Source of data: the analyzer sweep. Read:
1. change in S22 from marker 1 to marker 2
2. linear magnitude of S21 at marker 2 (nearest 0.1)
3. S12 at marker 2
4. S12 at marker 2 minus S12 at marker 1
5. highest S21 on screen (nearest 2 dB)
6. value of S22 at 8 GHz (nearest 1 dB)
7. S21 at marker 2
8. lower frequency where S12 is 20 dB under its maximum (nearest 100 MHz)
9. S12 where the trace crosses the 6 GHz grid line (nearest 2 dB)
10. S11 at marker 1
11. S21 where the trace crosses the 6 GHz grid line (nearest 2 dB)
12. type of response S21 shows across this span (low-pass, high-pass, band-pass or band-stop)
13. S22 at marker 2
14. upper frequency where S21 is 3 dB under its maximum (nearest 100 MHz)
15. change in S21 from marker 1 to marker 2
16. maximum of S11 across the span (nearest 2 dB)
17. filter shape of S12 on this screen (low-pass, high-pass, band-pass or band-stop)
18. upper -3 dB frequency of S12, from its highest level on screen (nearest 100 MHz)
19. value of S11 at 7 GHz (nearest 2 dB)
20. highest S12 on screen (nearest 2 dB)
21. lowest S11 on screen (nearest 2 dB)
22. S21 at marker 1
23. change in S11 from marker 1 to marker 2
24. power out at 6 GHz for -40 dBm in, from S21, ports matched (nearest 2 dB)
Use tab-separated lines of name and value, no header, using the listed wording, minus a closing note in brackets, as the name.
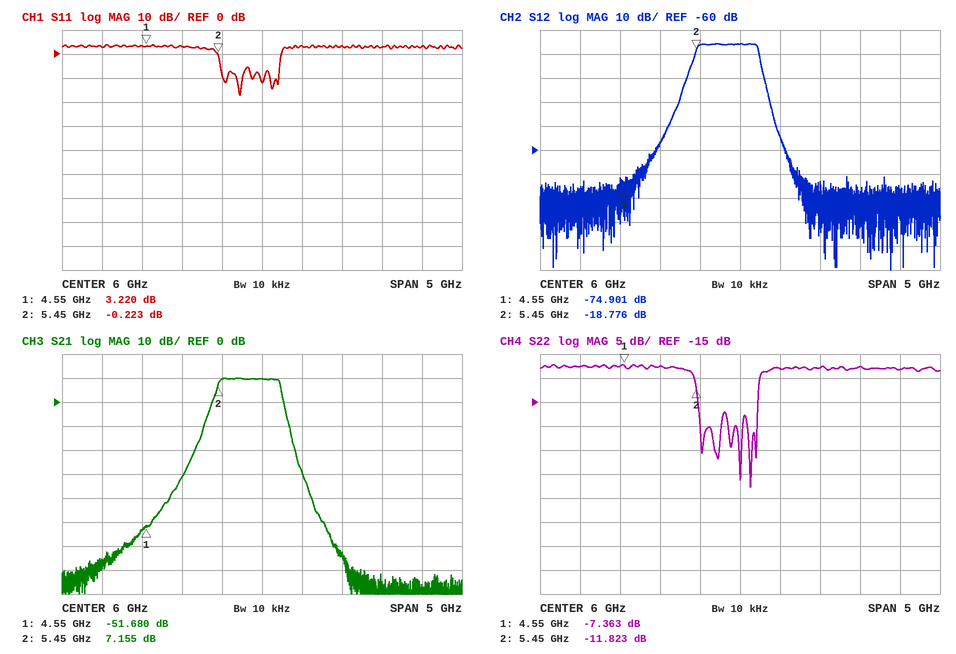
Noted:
change in S22 from marker 1 to marker 2	-4.460 dB
linear magnitude of S21 at marker 2	2.3
S12 at marker 2	-18.776 dB
S12 at marker 2 minus S12 at marker 1	56.125 dB
highest S21 on screen	10 dB
value of S22 at 8 GHz	-8 dB
S21 at marker 2	7.155 dB
lower frequency where S12 is 20 dB under its maximum	5.3 GHz
S12 where the trace crosses the 6 GHz grid line	-16 dB
S11 at marker 1	3.220 dB
S21 where the trace crosses the 6 GHz grid line	10 dB
type of response S21 shows across this span	band-pass
S22 at marker 2	-11.823 dB
upper frequency where S21 is 3 dB under its maximum	6.2 GHz
change in S21 from marker 1 to marker 2	58.835 dB
maximum of S11 across the span	4 dB
filter shape of S12 on this screen	band-pass
upper -3 dB frequency of S12, from its highest level on screen	6.2 GHz
value of S11 at 7 GHz	4 dB
highest S12 on screen	-16 dB
lowest S11 on screen	-18 dB
S21 at marker 1	-51.680 dB
change in S11 from marker 1 to marker 2	-3.443 dB
power out at 6 GHz for -40 dBm in, from S21, ports matched	-30 dBm
